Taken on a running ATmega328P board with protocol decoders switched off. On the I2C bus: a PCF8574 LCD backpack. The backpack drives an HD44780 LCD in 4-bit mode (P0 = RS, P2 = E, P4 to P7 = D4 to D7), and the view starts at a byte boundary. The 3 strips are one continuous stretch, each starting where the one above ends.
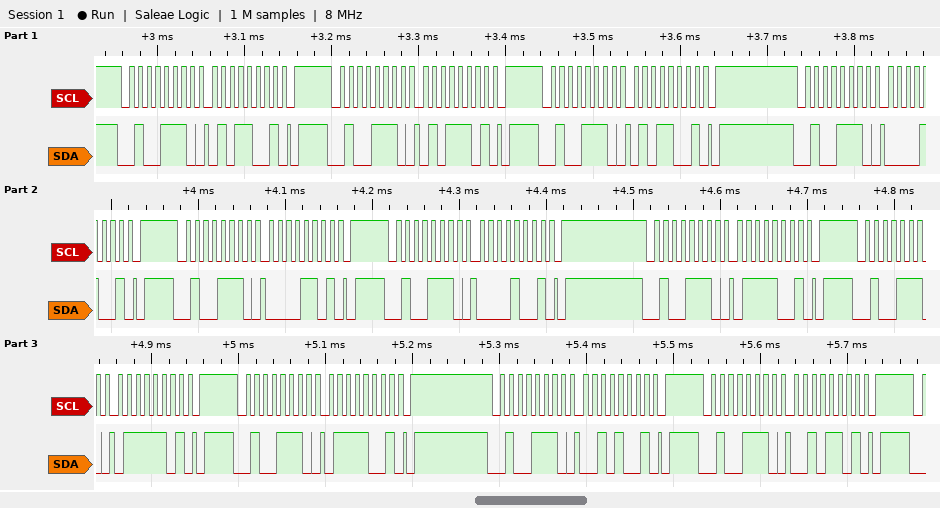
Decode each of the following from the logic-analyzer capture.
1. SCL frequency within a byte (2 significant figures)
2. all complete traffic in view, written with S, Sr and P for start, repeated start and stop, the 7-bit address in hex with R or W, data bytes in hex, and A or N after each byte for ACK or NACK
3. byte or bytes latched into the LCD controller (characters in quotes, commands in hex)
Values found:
100 kHz
S 27W A 59 A P S 27W A 5D A P S 27W A 59 A P S 27W A 09 A P S 27W A 0D A P S 27W A 09 A P S 27W A 79 A P S 27W A 7D A P S 27W A 79 A P S 27W A 29 A P S 27W A 2D A P
'P'
